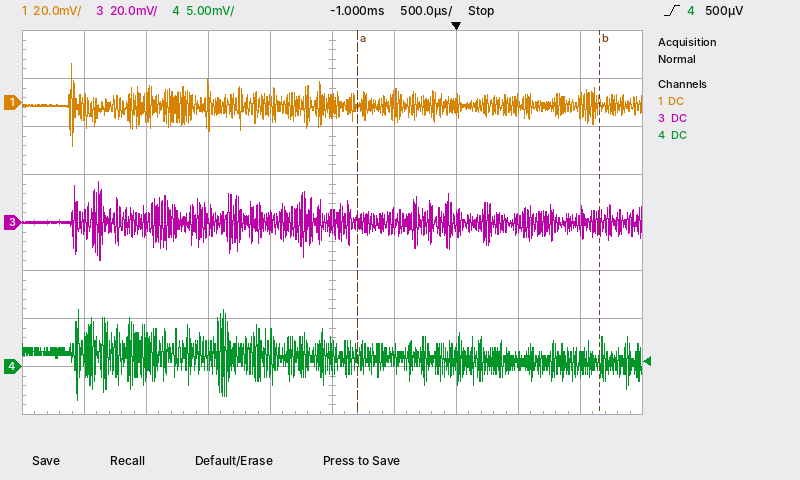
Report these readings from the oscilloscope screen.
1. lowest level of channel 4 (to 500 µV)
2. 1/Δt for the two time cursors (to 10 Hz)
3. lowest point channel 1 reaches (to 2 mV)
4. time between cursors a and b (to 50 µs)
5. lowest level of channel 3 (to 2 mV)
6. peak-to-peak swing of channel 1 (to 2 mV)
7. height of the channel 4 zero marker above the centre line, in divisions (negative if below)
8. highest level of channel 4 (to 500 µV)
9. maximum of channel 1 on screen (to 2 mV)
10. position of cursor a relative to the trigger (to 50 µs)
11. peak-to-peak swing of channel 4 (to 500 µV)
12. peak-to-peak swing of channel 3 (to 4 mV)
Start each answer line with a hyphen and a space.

- -3.5 mV
- 510 Hz
- -18 mV
- 1.95 ms
- -16 mV
- 34 mV
- -3.0 div
- 6.0 mV
- 16 mV
- -800 µs
- 9.5 mV
- 32 mV
